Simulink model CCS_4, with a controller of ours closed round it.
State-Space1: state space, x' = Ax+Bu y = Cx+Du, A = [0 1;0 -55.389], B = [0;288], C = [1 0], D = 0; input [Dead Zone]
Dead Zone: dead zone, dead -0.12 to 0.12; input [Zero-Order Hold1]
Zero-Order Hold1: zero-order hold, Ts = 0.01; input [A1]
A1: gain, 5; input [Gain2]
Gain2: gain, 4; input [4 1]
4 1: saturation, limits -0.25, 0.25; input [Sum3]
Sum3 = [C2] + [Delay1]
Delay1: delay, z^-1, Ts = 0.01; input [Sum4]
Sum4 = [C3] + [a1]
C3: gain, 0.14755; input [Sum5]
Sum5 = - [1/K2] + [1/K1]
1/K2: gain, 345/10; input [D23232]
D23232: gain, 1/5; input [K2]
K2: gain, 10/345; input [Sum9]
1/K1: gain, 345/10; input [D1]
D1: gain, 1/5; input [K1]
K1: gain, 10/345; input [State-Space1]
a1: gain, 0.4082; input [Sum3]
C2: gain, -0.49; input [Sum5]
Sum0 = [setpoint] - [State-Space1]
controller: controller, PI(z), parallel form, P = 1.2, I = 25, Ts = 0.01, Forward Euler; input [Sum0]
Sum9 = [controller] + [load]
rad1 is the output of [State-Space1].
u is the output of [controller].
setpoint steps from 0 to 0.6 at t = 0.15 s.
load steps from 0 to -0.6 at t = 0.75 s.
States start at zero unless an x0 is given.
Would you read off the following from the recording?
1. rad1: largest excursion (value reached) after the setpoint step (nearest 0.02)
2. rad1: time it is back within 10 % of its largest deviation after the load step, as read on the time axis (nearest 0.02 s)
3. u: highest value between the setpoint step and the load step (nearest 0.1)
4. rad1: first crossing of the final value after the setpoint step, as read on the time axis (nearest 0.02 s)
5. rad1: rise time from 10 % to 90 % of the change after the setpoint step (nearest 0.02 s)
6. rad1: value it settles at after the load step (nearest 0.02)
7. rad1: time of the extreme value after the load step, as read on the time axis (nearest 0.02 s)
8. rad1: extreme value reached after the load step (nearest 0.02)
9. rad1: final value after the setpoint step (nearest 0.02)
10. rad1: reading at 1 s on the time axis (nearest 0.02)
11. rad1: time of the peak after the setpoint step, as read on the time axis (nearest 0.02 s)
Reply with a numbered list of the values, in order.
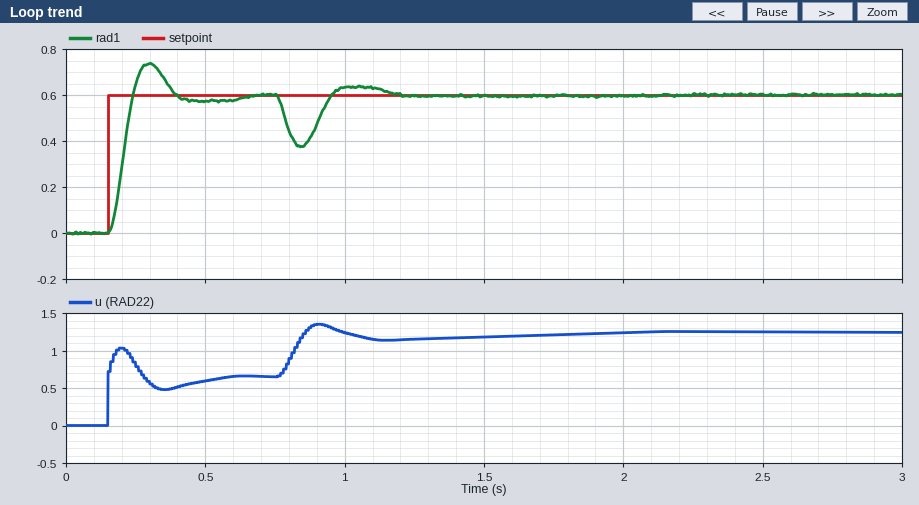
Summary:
1. 0.74
2. 1.14 s
3. 1.0
4. 0.24 s
5. 0.06 s
6. 0.60
7. 0.84 s
8. 0.38
9. 0.60
10. 0.64
11. 0.30 s
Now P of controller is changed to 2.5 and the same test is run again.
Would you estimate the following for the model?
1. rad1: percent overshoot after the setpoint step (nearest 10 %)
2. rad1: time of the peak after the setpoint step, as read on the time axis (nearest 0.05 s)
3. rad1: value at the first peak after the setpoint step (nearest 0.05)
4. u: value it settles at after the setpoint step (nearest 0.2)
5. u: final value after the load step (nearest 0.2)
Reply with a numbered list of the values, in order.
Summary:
1. 20 %
2. 0.25 s
3. 0.70
4. 0.6
5. 1.2
